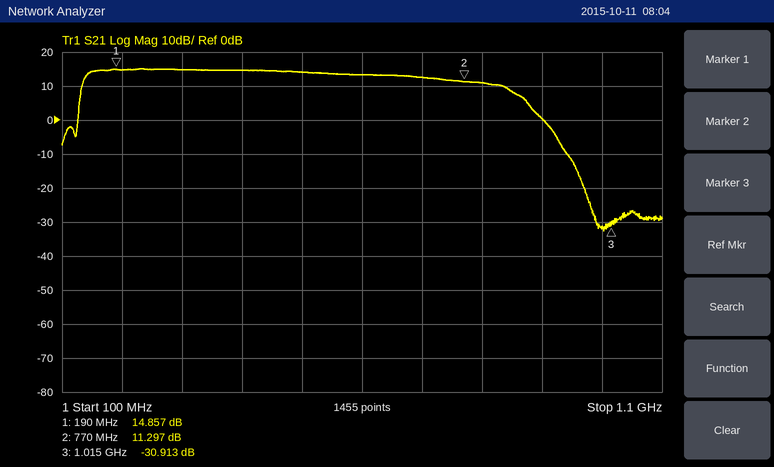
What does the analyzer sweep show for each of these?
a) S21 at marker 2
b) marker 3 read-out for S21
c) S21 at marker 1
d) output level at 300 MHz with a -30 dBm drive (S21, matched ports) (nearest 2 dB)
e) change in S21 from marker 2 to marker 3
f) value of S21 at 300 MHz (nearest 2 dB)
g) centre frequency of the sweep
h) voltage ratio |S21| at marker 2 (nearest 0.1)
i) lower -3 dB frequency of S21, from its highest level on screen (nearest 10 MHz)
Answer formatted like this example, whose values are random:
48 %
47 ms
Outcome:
11.297 dB
-30.913 dB
14.857 dB
-16 dBm
-42.210 dB
14 dB
600 MHz
3.7
140 MHz
